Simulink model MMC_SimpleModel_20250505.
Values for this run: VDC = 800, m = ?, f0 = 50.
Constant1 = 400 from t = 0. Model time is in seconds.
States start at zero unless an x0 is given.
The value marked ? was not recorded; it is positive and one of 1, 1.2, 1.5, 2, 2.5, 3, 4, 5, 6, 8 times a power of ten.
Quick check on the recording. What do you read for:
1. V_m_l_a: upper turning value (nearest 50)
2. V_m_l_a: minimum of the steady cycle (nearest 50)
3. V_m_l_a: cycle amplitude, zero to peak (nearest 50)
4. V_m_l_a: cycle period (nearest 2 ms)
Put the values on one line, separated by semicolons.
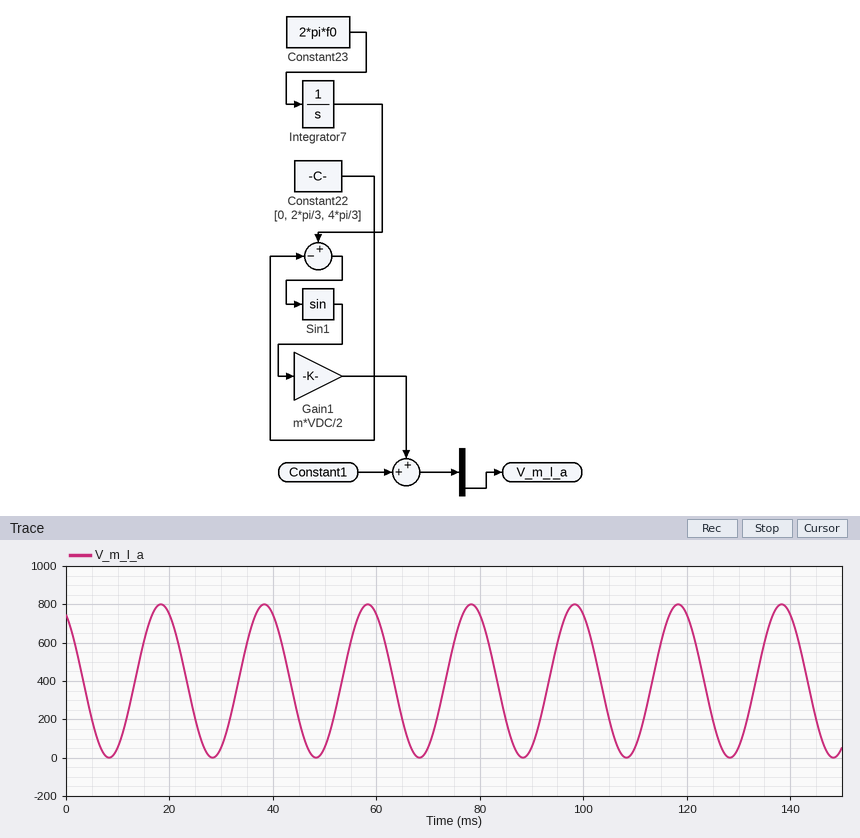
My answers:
800; 0; 400; 20 ms
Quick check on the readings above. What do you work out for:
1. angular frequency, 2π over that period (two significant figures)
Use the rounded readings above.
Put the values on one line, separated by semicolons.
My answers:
0.31 rad/ms
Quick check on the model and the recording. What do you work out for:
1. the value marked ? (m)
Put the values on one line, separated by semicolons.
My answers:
1
